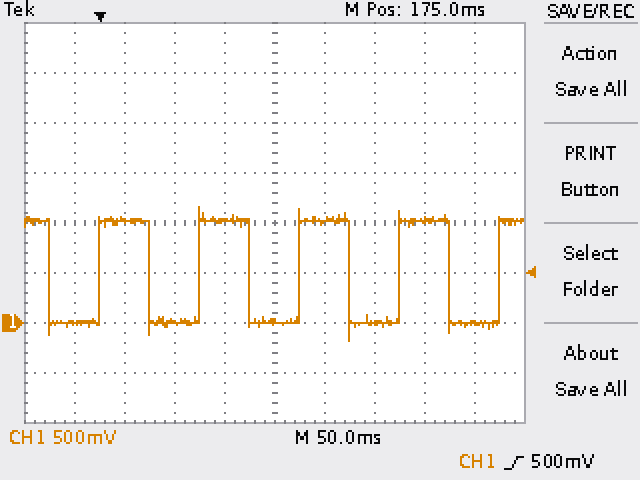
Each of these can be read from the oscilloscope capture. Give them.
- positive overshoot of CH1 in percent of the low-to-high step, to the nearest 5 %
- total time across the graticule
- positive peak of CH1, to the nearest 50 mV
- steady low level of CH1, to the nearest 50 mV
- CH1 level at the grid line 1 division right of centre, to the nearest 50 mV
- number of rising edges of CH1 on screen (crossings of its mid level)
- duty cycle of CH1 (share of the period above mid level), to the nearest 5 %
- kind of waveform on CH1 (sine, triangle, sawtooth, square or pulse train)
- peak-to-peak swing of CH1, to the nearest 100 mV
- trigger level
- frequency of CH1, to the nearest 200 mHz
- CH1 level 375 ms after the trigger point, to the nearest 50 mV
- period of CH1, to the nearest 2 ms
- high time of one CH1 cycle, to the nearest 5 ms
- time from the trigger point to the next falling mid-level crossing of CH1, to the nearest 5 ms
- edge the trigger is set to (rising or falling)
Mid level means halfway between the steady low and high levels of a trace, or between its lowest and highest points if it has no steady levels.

15 %
500 ms
1.15 V
0 mV
1.00 V
5
50 %
square
1.30 V
500 mV
10.0 Hz
0 mV
100 ms
50 ms
50 ms
rising
